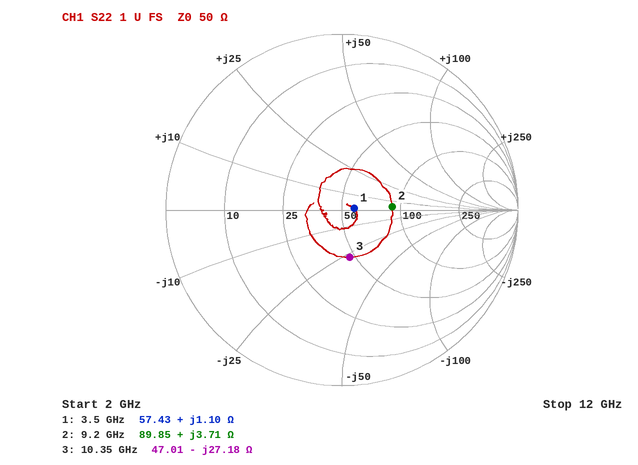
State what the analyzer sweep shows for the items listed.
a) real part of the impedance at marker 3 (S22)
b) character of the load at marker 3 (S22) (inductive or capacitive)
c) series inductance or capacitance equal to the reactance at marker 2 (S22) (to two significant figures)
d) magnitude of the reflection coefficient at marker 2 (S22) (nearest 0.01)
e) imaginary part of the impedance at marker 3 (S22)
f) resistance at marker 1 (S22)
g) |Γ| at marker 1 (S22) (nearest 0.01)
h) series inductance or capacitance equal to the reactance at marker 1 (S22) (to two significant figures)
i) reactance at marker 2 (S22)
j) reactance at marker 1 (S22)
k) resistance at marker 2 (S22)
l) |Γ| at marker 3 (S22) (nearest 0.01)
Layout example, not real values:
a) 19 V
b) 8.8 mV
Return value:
a) 47.01 Ω
b) capacitive
c) 64 pH
d) 0.29
e) -27.18 Ω
f) 57.43 Ω
g) 0.07
h) 50 pH
i) +3.71 Ω
j) +1.10 Ω
k) 89.85 Ω
l) 0.27
